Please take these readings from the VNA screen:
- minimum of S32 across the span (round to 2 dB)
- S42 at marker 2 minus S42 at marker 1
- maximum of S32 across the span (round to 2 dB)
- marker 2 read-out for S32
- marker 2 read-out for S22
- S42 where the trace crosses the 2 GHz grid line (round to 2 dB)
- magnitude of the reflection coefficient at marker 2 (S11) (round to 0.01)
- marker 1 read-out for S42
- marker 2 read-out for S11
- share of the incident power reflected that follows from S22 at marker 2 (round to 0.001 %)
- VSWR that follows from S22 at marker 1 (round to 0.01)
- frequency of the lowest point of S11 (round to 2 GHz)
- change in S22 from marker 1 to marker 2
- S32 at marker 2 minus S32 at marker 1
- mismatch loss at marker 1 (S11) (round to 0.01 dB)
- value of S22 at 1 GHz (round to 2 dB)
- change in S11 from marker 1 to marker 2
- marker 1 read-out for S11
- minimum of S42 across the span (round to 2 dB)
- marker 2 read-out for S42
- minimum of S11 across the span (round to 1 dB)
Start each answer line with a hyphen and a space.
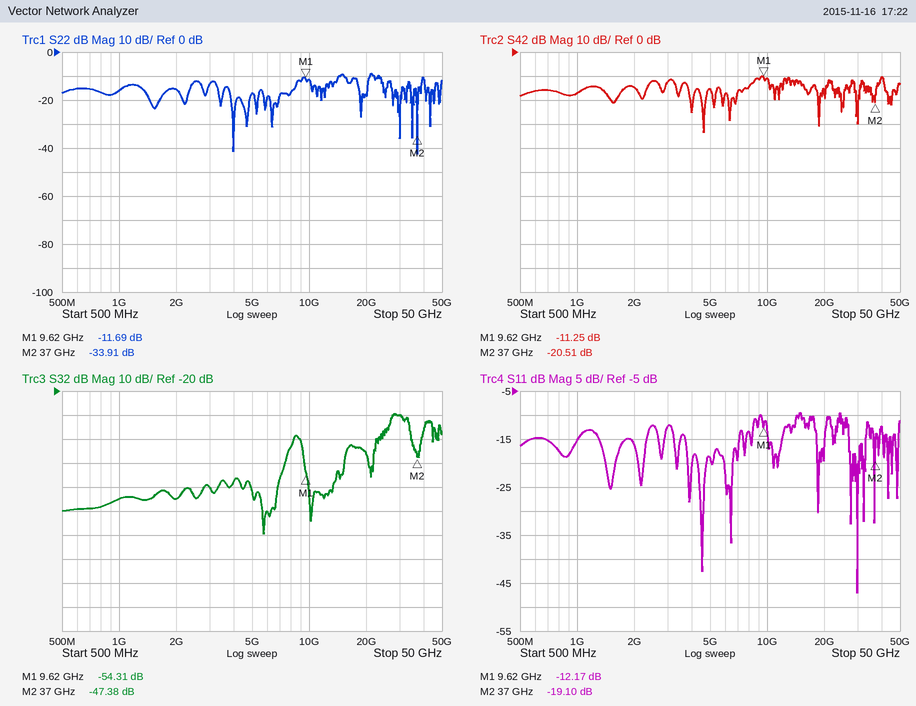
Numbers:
- -80 dB
- -9.26 dB
- -30 dB
- -47.38 dB
- -33.91 dB
- -14 dB
- 0.11
- -11.25 dB
- -19.10 dB
- 0.041 %
- 1.70
- 30 GHz
- -22.22 dB
- 6.93 dB
- 0.27 dB
- -16 dB
- -6.93 dB
- -12.17 dB
- -34 dB
- -20.51 dB
- -47 dB
